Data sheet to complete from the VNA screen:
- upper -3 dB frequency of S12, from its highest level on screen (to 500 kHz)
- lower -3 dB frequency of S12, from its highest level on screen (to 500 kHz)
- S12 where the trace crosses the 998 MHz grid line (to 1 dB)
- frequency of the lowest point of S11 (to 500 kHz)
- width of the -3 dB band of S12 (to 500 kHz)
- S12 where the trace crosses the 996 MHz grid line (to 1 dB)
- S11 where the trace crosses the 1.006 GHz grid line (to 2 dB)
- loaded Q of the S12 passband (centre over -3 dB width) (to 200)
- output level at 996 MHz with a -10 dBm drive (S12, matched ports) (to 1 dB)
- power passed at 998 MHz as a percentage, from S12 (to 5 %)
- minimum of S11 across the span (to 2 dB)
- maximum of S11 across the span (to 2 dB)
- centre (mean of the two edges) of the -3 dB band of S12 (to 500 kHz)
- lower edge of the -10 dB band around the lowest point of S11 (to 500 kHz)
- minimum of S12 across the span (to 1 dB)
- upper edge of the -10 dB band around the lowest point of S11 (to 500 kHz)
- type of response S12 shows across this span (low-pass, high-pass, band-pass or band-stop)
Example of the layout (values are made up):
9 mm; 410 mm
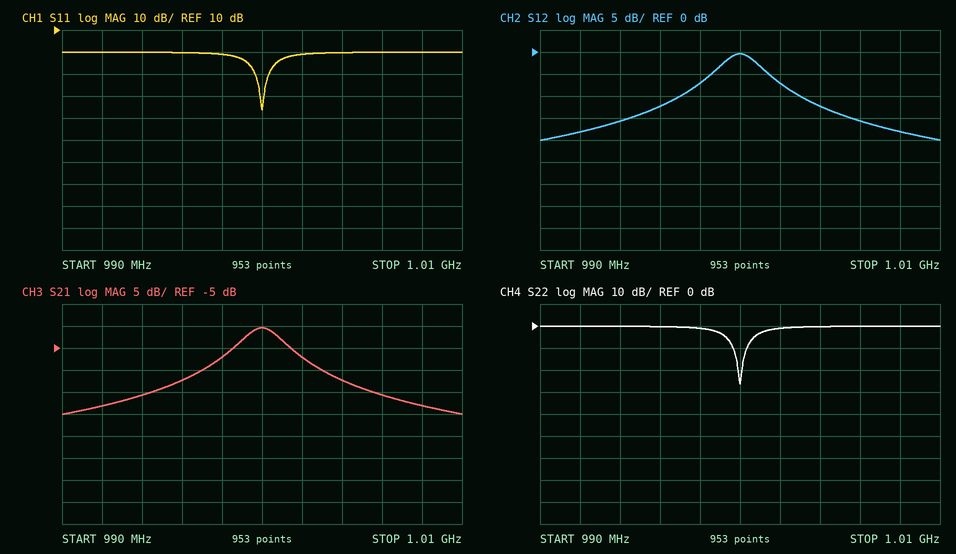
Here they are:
1.0010 GHz; 999.0 MHz; -7 dB; 1.0000 GHz; 2.0 MHz; -12 dB; 0 dB; 400; -22 dBm; 20 %; -26 dB; 0 dB; 1.0000 GHz; 999.5 MHz; -20 dB; 1.0005 GHz; band-pass
